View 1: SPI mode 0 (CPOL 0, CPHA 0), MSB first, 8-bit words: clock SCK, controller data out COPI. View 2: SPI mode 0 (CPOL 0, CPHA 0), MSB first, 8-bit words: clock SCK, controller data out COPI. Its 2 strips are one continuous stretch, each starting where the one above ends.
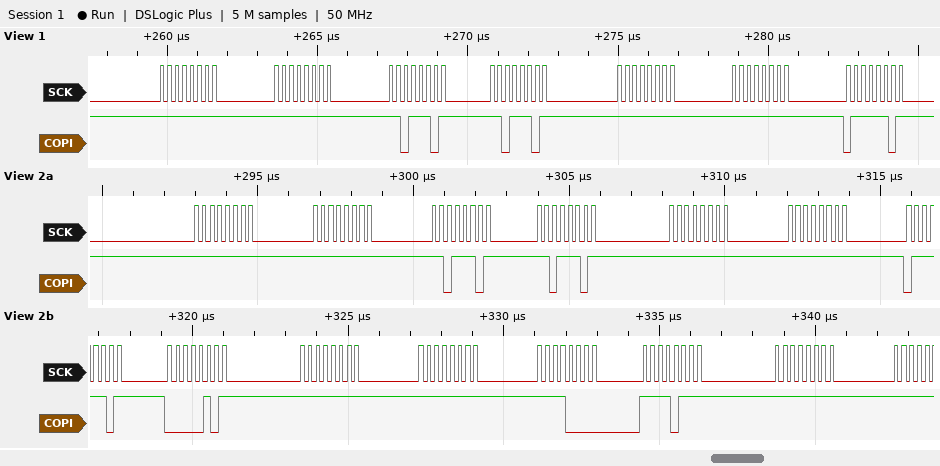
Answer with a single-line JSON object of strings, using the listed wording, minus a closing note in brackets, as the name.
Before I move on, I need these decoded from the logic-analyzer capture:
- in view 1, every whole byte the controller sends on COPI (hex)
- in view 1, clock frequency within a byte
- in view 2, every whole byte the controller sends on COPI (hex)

{"in view 1, every whole byte the controller sends on COPI": "0xFF 0xFF 0xDD 0xDD 0xFF 0xFF 0x7D", "in view 1, clock frequency within a byte": "4 MHz", "in view 2, every whole byte the controller sends on COPI": "0xFF 0xFF 0xDD 0xDD 0xFF 0xFF 0x7D 0x05 0xFF 0xFF 0xF0 0xF7 0xFF"}
